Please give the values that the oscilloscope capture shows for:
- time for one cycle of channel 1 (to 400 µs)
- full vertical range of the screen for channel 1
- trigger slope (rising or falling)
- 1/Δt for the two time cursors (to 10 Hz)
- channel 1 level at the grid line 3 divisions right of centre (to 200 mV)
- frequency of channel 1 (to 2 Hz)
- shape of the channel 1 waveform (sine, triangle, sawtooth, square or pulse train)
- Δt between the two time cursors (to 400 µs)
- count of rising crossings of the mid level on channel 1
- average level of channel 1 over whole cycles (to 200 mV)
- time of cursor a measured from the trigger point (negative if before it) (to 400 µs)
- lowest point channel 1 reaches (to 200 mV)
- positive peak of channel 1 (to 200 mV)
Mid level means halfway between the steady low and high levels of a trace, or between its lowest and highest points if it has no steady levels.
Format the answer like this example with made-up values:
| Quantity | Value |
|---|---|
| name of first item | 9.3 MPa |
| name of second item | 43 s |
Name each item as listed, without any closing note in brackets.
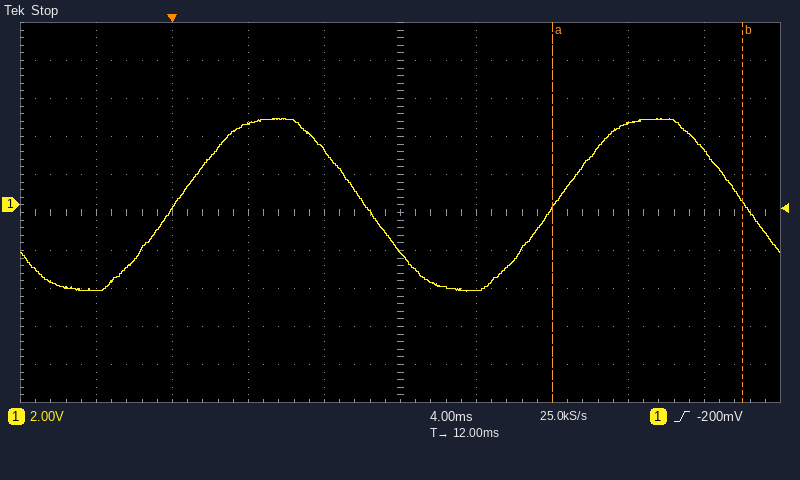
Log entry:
| Quantity | Value |
|---|---|
| time for one cycle of channel 1 | 20.0 ms |
| full vertical range of the screen for channel 1 | 20 V |
| trigger slope | rising |
| 1/Δt for the two time cursors | 100 Hz |
| channel 1 level at the grid line 3 divisions right of centre | 4.2 V |
| frequency of channel 1 | 50 Hz |
| shape of the channel 1 waveform | sine |
| Δt between the two time cursors | 10.0 ms |
| count of rising crossings of the mid level on channel 1 | 2 |
| average level of channel 1 over whole cycles | 0.0 V |
| time of cursor a measured from the trigger point (negative if before it) | +20.0 ms |
| lowest point channel 1 reaches | -4.6 V |
| positive peak of channel 1 | 4.6 V |
